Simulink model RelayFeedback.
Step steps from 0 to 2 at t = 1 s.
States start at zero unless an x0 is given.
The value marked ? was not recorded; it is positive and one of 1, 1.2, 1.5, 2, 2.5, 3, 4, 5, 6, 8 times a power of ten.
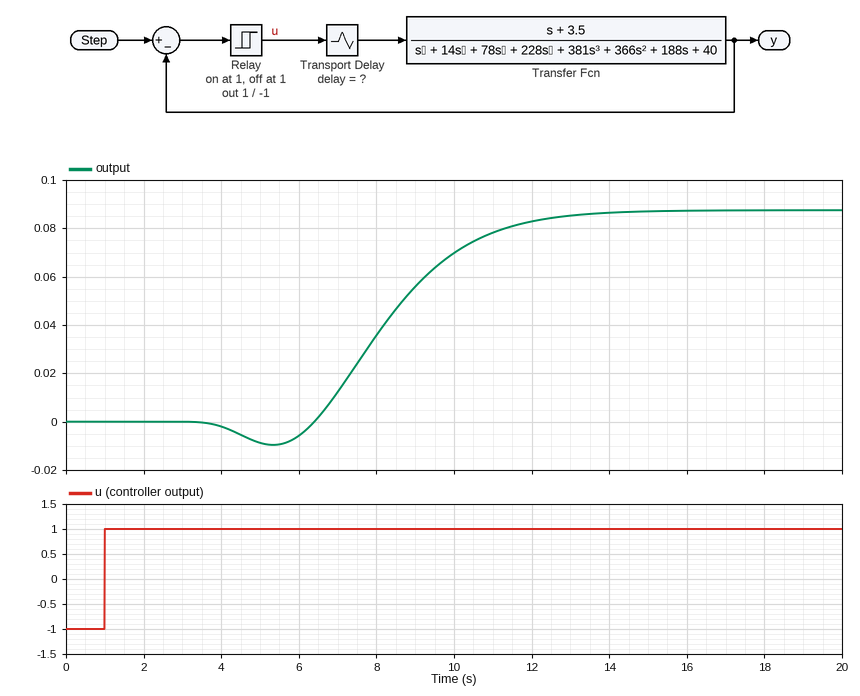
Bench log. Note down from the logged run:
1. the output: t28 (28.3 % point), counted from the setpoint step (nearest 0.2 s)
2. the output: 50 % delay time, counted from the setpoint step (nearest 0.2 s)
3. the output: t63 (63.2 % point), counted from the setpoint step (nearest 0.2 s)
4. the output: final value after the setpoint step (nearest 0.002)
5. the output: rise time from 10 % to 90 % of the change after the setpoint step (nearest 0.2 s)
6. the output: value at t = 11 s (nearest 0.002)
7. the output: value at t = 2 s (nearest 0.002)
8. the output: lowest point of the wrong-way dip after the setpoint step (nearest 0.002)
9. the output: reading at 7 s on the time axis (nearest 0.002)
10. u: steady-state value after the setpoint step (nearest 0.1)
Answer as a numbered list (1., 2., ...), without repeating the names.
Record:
1. 6.6 s
2. 7.4 s
3. 8.0 s
4. 0.088
5. 4.2 s
6. 0.078
7. 0.000
8. -0.010
9. 0.012
10. 1.0
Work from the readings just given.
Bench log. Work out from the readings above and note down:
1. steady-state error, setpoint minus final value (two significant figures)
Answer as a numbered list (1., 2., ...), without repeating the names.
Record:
1. 1.9
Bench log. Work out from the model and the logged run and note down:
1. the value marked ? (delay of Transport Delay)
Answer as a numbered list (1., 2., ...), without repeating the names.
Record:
1. 2.5
